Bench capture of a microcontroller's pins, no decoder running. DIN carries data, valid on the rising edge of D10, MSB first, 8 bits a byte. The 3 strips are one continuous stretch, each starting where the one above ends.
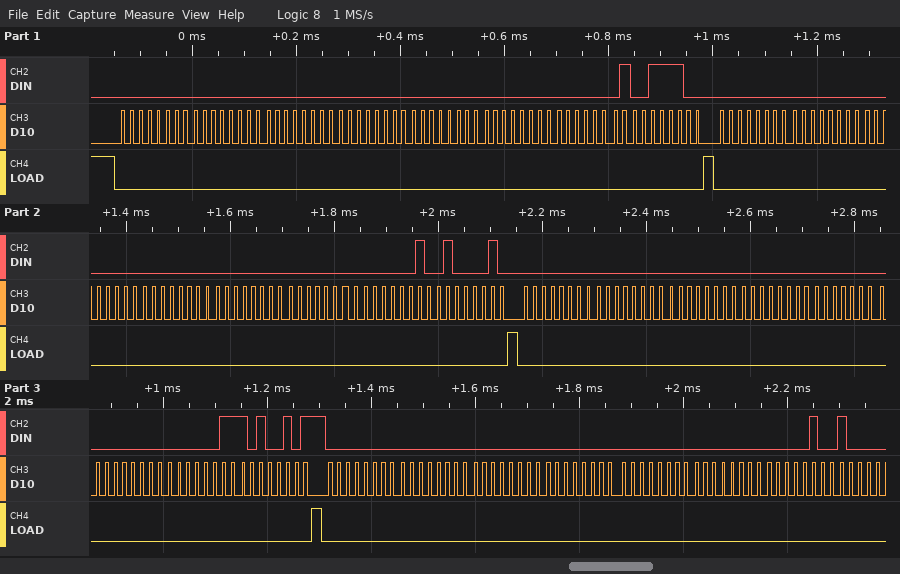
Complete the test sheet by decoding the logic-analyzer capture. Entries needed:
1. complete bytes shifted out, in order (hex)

0x00 0x00 0x00 0x00 0x00 0x00 0x01 0x3C 0x00 0x00 0x00 0x00 0x00 0x00 0x02 0x42 0x00 0x00 0x00 0x00 0x00 0x00 0x03 0xA5 0x00 0x00 0x00 0x00 0x00 0x00 0x04
